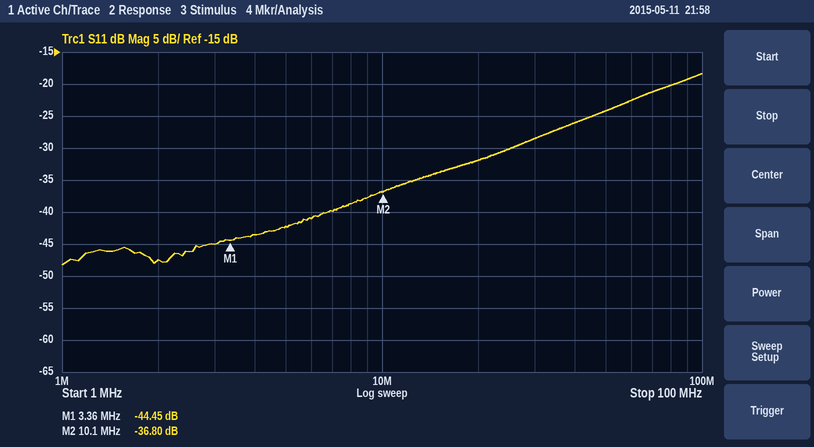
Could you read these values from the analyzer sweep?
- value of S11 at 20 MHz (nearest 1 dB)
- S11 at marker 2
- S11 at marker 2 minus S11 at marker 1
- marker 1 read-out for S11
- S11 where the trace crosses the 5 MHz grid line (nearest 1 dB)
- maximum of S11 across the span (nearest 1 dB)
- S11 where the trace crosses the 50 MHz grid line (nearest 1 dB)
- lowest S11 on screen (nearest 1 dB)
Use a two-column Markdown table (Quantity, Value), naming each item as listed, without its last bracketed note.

| Quantity | Value |
|---|---|
| value of S11 at 20 MHz | -32 dB |
| S11 at marker 2 | -36.80 dB |
| S11 at marker 2 minus S11 at marker 1 | 7.65 dB |
| marker 1 read-out for S11 | -44.45 dB |
| S11 where the trace crosses the 5 MHz grid line | -42 dB |
| maximum of S11 across the span | -18 dB |
| S11 where the trace crosses the 50 MHz grid line | -24 dB |
| lowest S11 on screen | -48 dB |
